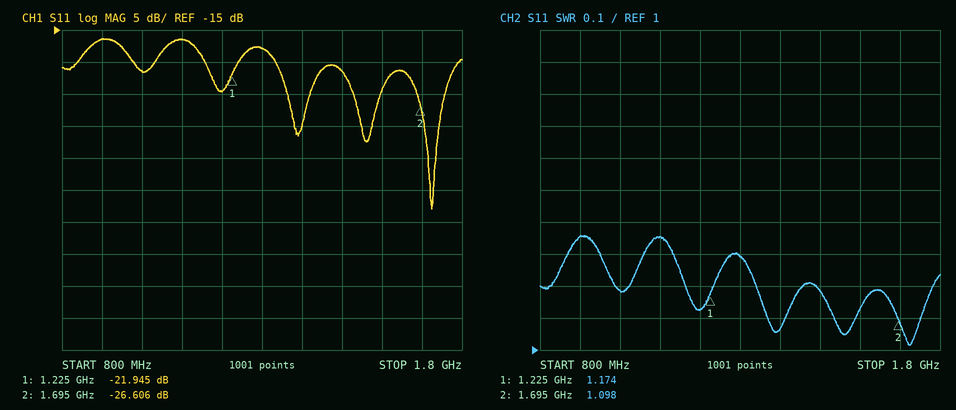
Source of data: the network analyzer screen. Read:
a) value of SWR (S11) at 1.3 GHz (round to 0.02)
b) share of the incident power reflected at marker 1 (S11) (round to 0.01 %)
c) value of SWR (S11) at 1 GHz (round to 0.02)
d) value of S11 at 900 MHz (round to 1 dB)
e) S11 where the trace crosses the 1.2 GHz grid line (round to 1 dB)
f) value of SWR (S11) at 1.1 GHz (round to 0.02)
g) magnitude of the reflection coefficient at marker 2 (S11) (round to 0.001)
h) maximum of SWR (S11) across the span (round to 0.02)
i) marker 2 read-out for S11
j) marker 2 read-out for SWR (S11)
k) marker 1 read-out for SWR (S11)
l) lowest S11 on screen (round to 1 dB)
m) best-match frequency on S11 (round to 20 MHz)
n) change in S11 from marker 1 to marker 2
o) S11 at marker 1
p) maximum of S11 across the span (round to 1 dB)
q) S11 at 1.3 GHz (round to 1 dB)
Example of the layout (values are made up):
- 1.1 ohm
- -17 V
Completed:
- 1.30
- 0.64 %
- 1.18
- -16 dB
- -25 dB
- 1.36
- 0.047
- 1.36
- -26.606 dB
- 1.098
- 1.174
- -43 dB
- 1.72 GHz
- -4.661 dB
- -21.945 dB
- -16 dB
- -18 dB
